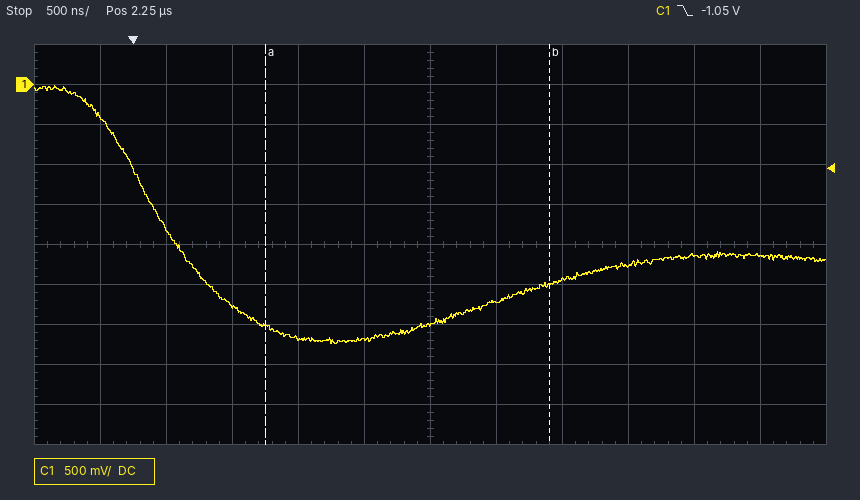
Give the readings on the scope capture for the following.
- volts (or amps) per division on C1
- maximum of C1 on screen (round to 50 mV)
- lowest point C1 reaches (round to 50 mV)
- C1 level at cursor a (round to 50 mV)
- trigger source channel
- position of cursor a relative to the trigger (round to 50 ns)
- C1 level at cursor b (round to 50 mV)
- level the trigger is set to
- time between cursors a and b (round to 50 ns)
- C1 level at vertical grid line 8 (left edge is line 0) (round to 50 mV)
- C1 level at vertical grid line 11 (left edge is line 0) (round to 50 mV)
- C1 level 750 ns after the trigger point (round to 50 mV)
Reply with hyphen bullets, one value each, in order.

- 500 mV
- 0 mV
- -3.25 V
- -3.00 V
- C1
- +1.00 µs
- -2.50 V
- -1.05 V
- 2.15 µs
- -2.45 V
- -2.15 V
- -2.75 V
